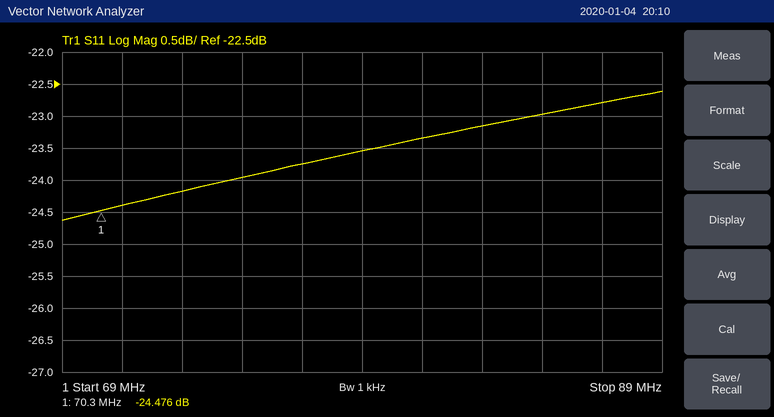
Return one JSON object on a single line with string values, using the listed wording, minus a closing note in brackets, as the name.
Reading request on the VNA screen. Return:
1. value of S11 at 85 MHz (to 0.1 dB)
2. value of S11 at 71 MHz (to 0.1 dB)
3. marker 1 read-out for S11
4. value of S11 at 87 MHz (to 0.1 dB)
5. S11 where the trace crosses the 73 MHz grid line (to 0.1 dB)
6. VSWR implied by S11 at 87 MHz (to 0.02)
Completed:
{"value of S11 at 85 MHz": "-23.0 dB", "value of S11 at 71 MHz": "-24.4 dB", "marker 1 read-out for S11": "-24.476 dB", "value of S11 at 87 MHz": "-22.8 dB", "S11 where the trace crosses the 73 MHz grid line": "-24.2 dB", "VSWR implied by S11 at 87 MHz": "1.16"}
